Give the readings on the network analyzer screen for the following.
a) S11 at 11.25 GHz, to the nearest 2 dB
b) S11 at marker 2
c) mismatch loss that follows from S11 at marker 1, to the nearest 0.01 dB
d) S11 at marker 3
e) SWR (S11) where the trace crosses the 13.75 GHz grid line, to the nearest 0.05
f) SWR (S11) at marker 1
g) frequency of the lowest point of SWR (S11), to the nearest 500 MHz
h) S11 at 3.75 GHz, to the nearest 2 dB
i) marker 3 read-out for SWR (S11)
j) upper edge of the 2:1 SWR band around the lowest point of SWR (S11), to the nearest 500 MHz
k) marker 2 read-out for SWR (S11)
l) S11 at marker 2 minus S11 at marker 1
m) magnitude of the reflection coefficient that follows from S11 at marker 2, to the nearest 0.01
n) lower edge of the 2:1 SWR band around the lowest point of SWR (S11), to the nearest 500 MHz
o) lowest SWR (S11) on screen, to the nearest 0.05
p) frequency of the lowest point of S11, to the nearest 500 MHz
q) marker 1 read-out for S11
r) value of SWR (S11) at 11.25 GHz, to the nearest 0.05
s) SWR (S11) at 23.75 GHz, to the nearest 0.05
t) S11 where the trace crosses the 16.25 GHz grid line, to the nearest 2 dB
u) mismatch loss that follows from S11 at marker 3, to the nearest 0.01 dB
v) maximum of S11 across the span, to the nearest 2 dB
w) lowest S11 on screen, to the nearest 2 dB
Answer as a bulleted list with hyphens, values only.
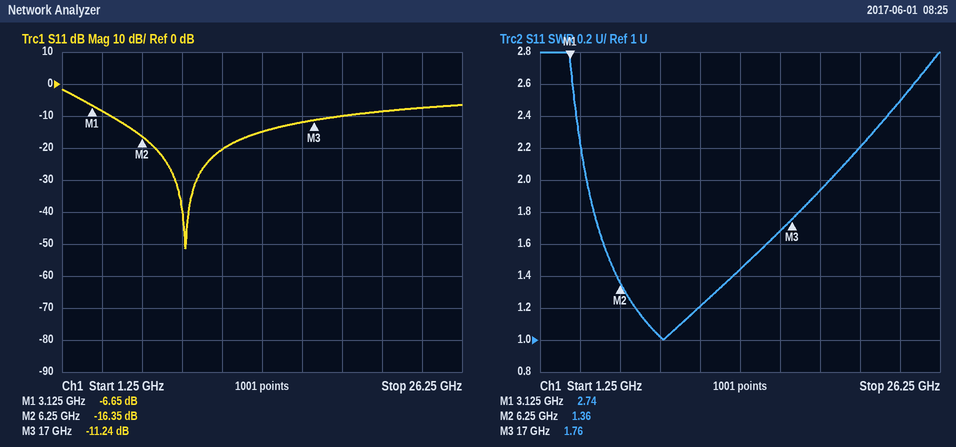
- -20 dB
- -16.35 dB
- 1.06 dB
- -11.24 dB
- 1.45
- 2.74
- 9.0 GHz
- -8 dB
- 1.76
- 19.5 GHz
- 1.36
- -9.70 dB
- 0.15
- 4.0 GHz
- 1.00
- 9.0 GHz
- -6.65 dB
- 1.20
- 2.50
- -12 dB
- 0.34 dB
- -2 dB
- -52 dB
